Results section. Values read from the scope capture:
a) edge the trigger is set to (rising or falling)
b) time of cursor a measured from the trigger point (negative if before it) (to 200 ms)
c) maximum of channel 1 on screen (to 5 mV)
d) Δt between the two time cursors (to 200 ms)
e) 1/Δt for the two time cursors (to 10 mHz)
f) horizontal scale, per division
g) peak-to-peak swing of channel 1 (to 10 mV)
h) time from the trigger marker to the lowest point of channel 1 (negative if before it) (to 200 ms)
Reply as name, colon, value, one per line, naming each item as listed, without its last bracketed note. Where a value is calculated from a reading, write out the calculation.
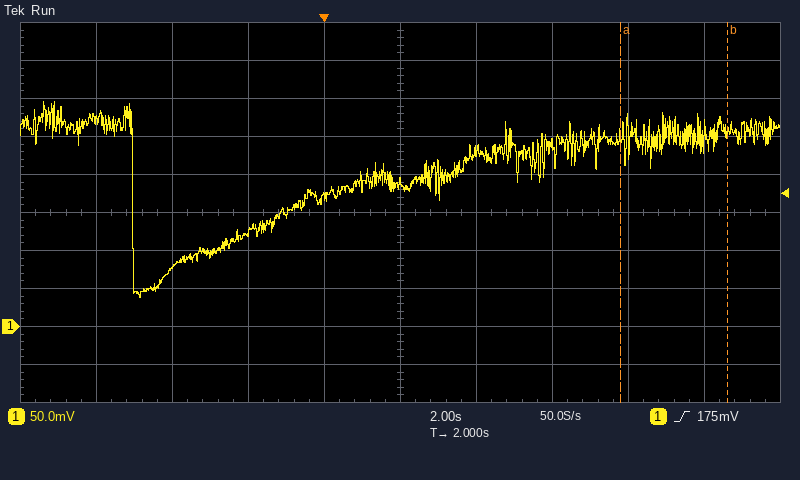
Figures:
edge the trigger is set to: rising
time of cursor a measured from the trigger point (negative if before it): +7.8 s
maximum of channel 1 on screen: 295 mV
Δt between the two time cursors: 2.8 s
1/Δt for the two time cursors: 1 / 2.8 s ≈ 360 mHz
horizontal scale, per division: 2 s
peak-to-peak swing of channel 1: 260 mV
time from the trigger marker to the lowest point of channel 1 (negative if before it): -4.8 s
